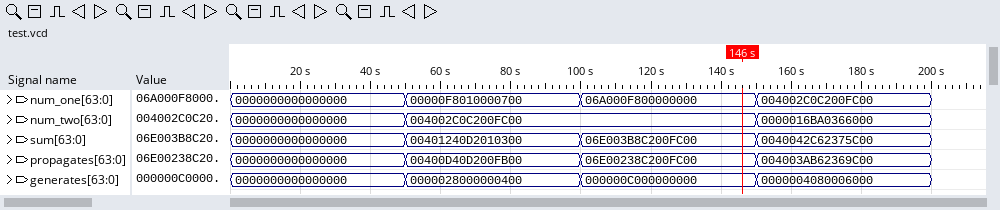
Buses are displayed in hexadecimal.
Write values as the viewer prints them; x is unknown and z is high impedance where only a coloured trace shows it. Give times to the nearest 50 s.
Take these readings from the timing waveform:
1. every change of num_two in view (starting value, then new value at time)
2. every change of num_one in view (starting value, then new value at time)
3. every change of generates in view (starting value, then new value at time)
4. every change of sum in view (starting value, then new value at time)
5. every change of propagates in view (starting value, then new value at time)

0000000000000000, 004002C0C200FC00 at 50 s, 0000016BA0366000 at 150 s
0000000000000000, 00000F8010000700 at 50 s, 06A000F800000000 at 100 s, 004002C0C200FC00 at 150 s
0000000000000000, 0000028000000400 at 50 s, 000000C000000000 at 100 s, 0000004080006000 at 150 s
0000000000000000, 00401240D2010300 at 50 s, 06E003B8C200FC00 at 100 s, 0040042C62375C00 at 150 s
0000000000000000, 00400D40D200FB00 at 50 s, 06E00238C200FC00 at 100 s, 004003AB62369C00 at 150 s
